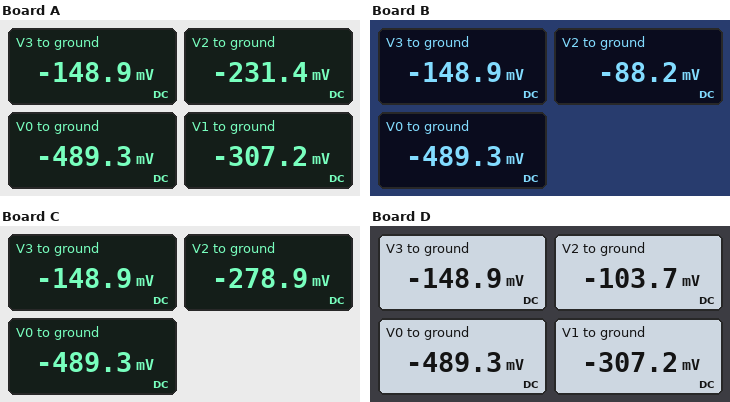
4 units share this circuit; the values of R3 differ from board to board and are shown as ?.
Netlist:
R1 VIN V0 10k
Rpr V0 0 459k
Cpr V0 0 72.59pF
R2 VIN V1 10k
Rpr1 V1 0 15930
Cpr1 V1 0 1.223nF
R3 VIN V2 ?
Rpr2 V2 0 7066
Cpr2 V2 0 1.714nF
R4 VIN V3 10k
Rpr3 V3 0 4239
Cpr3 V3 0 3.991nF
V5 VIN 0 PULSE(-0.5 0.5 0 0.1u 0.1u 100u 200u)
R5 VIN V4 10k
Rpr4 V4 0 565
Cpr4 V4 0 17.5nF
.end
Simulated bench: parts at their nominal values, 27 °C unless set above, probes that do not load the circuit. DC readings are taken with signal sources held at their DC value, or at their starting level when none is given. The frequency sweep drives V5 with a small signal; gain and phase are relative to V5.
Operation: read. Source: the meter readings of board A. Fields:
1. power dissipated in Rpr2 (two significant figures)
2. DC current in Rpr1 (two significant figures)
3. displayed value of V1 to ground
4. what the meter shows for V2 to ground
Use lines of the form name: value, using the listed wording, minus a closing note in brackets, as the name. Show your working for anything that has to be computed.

power dissipated in Rpr2: (0 V - (-231.4 mV))^2 / 7.066 kΩ = 7.6 µW
DC current in Rpr1: (0 V - (-307.2 mV)) / 15.93 kΩ = 19 µA
displayed value of V1 to ground: -307.2 mV
what the meter shows for V2 to ground: -231.4 mV
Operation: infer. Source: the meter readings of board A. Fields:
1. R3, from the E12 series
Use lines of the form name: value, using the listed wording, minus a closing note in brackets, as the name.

R3, from the E12 series: 8.2 kΩ
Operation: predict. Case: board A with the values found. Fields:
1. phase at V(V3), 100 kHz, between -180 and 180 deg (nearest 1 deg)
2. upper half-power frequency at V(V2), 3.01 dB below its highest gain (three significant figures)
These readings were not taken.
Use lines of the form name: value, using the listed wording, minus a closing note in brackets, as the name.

phase at V(V3), 100 kHz, between -180 and 180 deg: -82 deg
upper half-power frequency at V(V2), 3.01 dB below its highest gain: 24.5 kHz
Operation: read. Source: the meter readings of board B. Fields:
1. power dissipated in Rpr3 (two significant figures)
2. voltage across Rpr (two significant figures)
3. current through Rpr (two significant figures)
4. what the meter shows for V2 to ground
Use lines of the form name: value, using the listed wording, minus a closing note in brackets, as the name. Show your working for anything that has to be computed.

power dissipated in Rpr3: (0 V - (-148.9 mV))^2 / 4.239 kΩ = 5.2 µW
voltage across Rpr: 0 V - (-489.3 mV) = 490 mV
current through Rpr: (0 V - (-489.3 mV)) / 459 kΩ = 1.1 µA
what the meter shows for V2 to ground: -88.2 mV
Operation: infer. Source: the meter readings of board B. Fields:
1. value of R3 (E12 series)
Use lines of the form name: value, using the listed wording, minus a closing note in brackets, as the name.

value of R3: 33 kΩ
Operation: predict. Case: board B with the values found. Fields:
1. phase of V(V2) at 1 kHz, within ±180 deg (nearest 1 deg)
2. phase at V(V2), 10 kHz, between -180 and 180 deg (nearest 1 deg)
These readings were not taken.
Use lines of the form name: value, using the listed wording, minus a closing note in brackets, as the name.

phase of V(V2) at 1 kHz, within ±180 deg: -4 deg
phase at V(V2), 10 kHz, between -180 and 180 deg: -32 deg
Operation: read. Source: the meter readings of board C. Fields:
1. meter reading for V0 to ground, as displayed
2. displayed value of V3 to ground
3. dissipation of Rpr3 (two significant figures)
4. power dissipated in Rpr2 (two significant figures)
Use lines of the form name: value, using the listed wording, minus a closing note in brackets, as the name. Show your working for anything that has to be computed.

meter reading for V0 to ground, as displayed: -489.3 mV
displayed value of V3 to ground: -148.9 mV
dissipation of Rpr3: (0 V - (-148.9 mV))^2 / 4.239 kΩ = 5.2 µW
power dissipated in Rpr2: (0 V - (-278.9 mV))^2 / 7.066 kΩ = 11 µW
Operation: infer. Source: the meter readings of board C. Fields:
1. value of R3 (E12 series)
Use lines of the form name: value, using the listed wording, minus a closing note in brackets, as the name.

value of R3: 5.6 kΩ
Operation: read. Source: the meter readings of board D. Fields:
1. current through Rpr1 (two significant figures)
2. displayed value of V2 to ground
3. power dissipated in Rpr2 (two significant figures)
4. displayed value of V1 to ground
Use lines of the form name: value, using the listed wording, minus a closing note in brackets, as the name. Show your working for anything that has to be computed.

current through Rpr1: (0 V - (-307.2 mV)) / 15.93 kΩ = 19 µA
displayed value of V2 to ground: -103.7 mV
power dissipated in Rpr2: (0 V - (-103.7 mV))^2 / 7.066 kΩ = 1.5 µW
displayed value of V1 to ground: -307.2 mV
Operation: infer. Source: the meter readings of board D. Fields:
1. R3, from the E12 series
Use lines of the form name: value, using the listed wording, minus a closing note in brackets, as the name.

R3, from the E12 series: 27 kΩ
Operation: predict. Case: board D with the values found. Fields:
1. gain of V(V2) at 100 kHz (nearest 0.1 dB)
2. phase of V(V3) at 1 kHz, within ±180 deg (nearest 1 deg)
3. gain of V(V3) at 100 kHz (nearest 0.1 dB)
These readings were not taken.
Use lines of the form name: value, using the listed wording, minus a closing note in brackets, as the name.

gain of V(V2) at 100 kHz: -29.4 dB
phase of V(V3) at 1 kHz, within ±180 deg: -4 deg
gain of V(V3) at 100 kHz: -28.1 dB
